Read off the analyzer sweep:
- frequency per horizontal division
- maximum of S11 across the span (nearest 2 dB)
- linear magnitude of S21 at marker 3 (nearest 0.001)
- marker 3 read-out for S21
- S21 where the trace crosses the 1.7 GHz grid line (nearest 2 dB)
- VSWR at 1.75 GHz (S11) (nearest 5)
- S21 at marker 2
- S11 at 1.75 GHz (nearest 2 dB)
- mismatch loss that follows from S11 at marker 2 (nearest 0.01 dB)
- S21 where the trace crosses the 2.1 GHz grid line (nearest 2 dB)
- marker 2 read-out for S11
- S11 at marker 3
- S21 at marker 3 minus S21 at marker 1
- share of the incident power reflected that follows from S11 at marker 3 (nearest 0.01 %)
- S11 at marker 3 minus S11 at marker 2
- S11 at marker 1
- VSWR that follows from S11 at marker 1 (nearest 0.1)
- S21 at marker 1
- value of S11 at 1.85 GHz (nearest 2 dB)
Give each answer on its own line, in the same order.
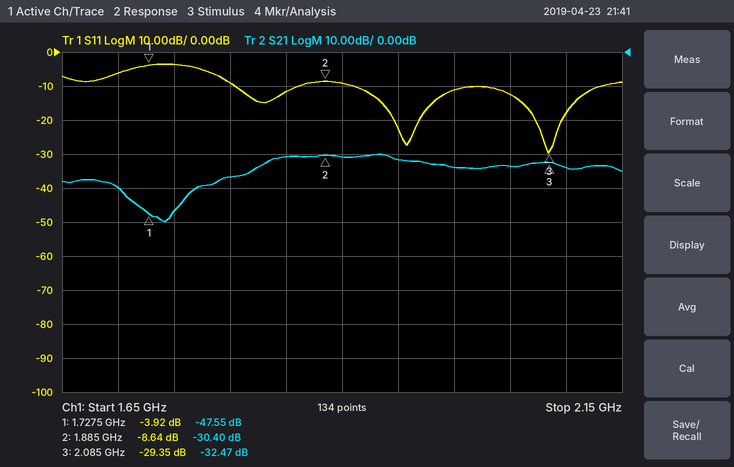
50 MHz
-4 dB
0.024
-32.47 dB
-40 dB
5
-30.40 dB
-4 dB
0.64 dB
-34 dB
-8.64 dB
-29.35 dB
15.08 dB
0.12 %
-20.71 dB
-3.92 dB
4.5
-47.55 dB
-12 dB
